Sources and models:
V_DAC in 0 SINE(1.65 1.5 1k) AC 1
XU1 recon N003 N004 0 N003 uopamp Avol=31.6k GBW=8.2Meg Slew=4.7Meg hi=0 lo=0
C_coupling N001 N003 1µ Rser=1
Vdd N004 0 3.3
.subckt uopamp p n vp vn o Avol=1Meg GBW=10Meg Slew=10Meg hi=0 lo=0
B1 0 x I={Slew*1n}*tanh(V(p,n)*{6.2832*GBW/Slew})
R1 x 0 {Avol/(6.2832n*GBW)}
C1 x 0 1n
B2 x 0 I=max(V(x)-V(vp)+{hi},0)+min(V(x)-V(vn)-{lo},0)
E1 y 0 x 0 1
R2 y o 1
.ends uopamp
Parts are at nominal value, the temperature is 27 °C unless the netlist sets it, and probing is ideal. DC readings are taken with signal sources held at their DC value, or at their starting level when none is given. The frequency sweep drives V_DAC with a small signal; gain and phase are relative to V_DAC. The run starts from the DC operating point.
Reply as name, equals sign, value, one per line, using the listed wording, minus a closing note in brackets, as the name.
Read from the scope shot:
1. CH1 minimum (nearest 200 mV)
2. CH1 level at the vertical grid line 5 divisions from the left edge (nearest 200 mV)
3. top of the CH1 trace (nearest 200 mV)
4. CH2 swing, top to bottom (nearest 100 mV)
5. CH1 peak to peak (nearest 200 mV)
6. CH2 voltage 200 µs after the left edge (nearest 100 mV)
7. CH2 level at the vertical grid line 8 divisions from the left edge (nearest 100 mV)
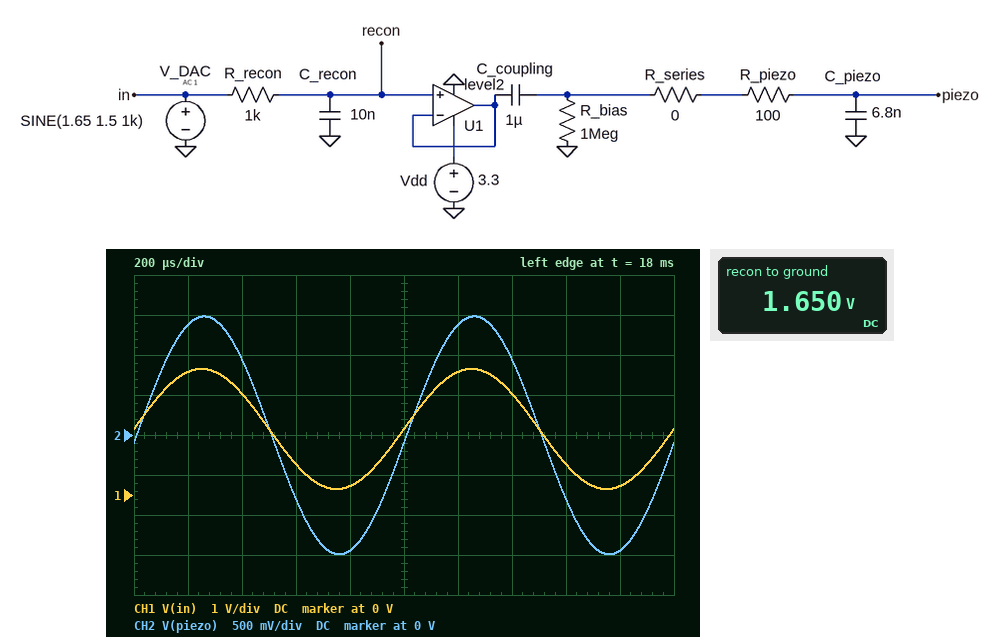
CH1 minimum = 200 mV
CH1 level at the vertical grid line 5 divisions from the left edge = 1.6 V
top of the CH1 trace = 3.2 V
CH2 swing, top to bottom = 3.0 V
CH1 peak to peak = 3.0 V
CH2 voltage 200 µs after the left edge = 1.4 V
CH2 level at the vertical grid line 8 divisions from the left edge = -800 mV
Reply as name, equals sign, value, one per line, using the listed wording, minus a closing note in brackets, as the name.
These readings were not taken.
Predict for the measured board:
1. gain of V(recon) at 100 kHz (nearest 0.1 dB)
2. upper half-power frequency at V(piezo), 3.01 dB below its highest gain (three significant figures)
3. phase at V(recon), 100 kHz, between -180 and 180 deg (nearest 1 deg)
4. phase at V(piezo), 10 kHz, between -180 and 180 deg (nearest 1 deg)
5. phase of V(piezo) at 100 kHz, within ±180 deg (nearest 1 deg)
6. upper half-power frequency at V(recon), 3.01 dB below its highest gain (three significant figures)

gain of V(recon) at 100 kHz = -16.1 dB
upper half-power frequency at V(piezo), 3.01 dB below its highest gain = 15.8 kHz
phase at V(recon), 100 kHz, between -180 and 180 deg = -81 deg
phase at V(piezo), 10 kHz, between -180 and 180 deg = -35 deg
phase of V(piezo) at 100 kHz, within ±180 deg = -105 deg
upper half-power frequency at V(recon), 3.01 dB below its highest gain = 15.9 kHz
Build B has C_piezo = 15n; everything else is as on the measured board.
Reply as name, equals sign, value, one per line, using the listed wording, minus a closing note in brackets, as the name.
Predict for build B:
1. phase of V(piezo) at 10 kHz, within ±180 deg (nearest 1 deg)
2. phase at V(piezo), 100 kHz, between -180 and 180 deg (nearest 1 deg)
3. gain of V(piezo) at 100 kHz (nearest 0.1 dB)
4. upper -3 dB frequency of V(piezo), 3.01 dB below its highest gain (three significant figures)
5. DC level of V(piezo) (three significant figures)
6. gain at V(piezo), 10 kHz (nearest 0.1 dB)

phase of V(piezo) at 10 kHz, within ±180 deg = -37 deg
phase at V(piezo), 100 kHz, between -180 and 180 deg = -125 deg
gain of V(piezo) at 100 kHz = -18.9 dB
upper -3 dB frequency of V(piezo), 3.01 dB below its highest gain = 15.6 kHz
DC level of V(piezo) = 1.62 V
gain at V(piezo), 10 kHz = -1.6 dB
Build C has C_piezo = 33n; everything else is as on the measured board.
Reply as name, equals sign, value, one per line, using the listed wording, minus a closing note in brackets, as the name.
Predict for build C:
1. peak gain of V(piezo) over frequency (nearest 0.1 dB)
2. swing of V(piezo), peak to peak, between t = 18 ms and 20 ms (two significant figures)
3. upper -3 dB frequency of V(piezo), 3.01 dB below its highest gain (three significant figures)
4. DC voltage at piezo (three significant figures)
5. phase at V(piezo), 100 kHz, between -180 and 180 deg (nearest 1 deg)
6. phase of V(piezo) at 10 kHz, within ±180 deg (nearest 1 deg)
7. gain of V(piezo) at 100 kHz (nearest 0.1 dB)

peak gain of V(piezo) over frequency = -0.3 dB
swing of V(piezo), peak to peak, between t = 18 ms and 20 ms = 2.9 V
upper -3 dB frequency of V(piezo), 3.01 dB below its highest gain = 14.6 kHz
DC voltage at piezo = 1.52 V
phase at V(piezo), 100 kHz, between -180 and 180 deg = -145 deg
phase of V(piezo) at 10 kHz, within ±180 deg = -44 deg
gain of V(piezo) at 100 kHz = -23.4 dB
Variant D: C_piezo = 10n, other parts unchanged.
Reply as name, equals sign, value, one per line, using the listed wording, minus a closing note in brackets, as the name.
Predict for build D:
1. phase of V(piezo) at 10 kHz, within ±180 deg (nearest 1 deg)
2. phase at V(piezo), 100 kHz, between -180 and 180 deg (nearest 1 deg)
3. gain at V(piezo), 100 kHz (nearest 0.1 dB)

phase of V(piezo) at 10 kHz, within ±180 deg = -36 deg
phase at V(piezo), 100 kHz, between -180 and 180 deg = -114 deg
gain at V(piezo), 100 kHz = -17.6 dB
